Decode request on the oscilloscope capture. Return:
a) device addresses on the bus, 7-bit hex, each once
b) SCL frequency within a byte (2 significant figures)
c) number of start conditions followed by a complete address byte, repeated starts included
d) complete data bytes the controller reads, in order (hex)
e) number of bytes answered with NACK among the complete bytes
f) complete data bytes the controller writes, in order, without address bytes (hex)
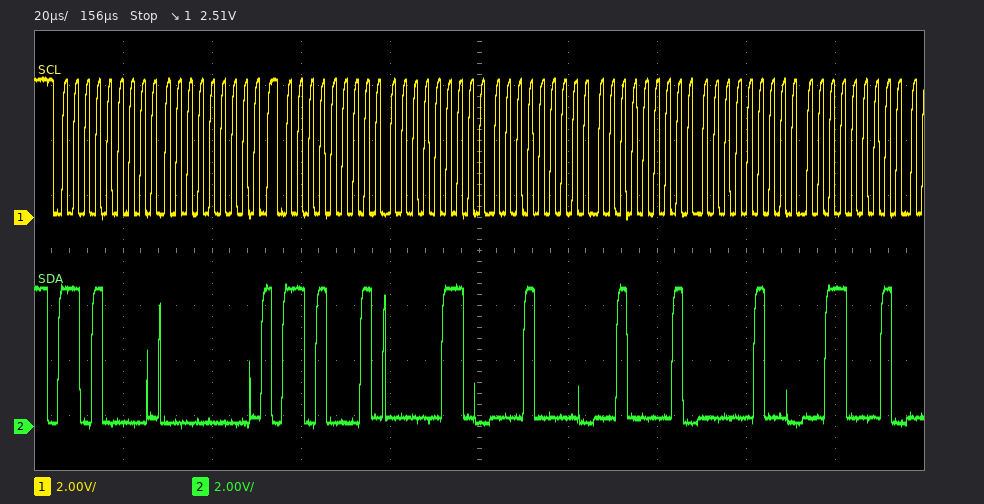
0x68
400 kHz
2
06 10 21 04 31
0
00
